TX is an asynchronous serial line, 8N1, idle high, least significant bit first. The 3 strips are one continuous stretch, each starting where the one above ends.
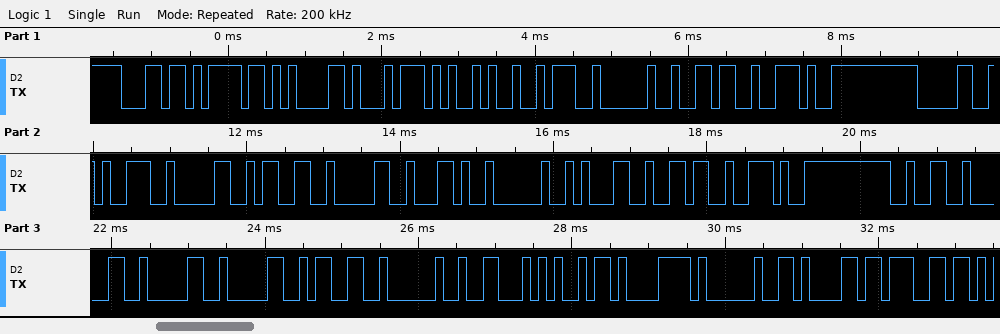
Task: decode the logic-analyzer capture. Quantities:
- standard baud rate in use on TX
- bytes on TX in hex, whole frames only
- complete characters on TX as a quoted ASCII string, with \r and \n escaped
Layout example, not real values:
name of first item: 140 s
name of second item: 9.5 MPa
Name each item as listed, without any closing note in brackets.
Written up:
standard baud rate in use on TX: 9600 baud
bytes on TX in hex, whole frames only: 6C 6F 61 74 29 3A 20 36 2E 30 39 30 33 30 2C 20 31 36 2E 32 30 30 30 33 20 46 69 78 20 61 67
complete characters on TX as a quoted ASCII string, with \r and \n escaped: "loat): 6.09030, 16.20003 Fix ag"
